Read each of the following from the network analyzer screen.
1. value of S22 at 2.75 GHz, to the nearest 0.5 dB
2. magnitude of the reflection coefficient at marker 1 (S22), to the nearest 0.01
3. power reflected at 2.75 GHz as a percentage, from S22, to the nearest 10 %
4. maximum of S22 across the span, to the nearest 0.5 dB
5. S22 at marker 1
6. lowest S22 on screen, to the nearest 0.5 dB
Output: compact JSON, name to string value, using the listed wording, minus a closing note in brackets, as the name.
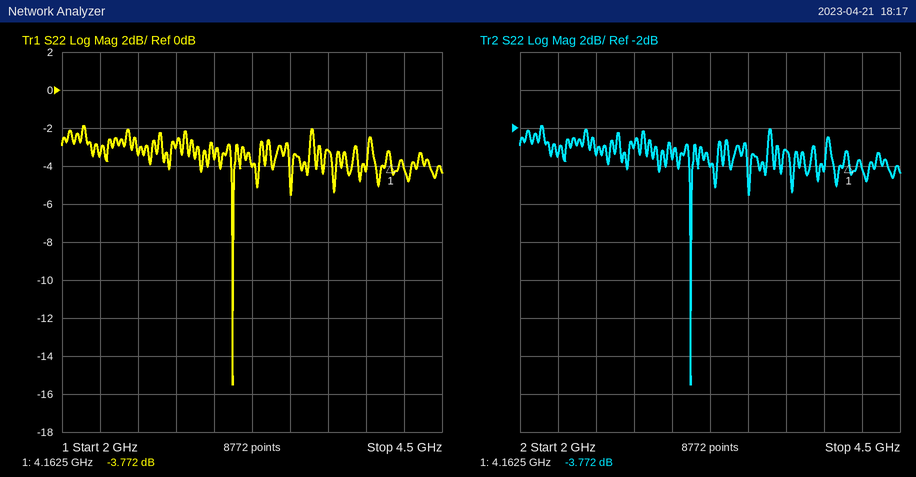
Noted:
{"value of S22 at 2.75 GHz, to the nearest 0.5 dB": "-3.0 dB", "magnitude of the reflection coefficient at marker 1 (S22), to the nearest 0.01": "0.65", "power reflected at 2.75 GHz as a percentage, from S22, to the nearest 10 %": "50 %", "maximum of S22 across the span, to the nearest 0.5 dB": "-2.0 dB", "S22 at marker 1": "-3.772 dB", "lowest S22 on screen, to the nearest 0.5 dB": "-15.5 dB"}
